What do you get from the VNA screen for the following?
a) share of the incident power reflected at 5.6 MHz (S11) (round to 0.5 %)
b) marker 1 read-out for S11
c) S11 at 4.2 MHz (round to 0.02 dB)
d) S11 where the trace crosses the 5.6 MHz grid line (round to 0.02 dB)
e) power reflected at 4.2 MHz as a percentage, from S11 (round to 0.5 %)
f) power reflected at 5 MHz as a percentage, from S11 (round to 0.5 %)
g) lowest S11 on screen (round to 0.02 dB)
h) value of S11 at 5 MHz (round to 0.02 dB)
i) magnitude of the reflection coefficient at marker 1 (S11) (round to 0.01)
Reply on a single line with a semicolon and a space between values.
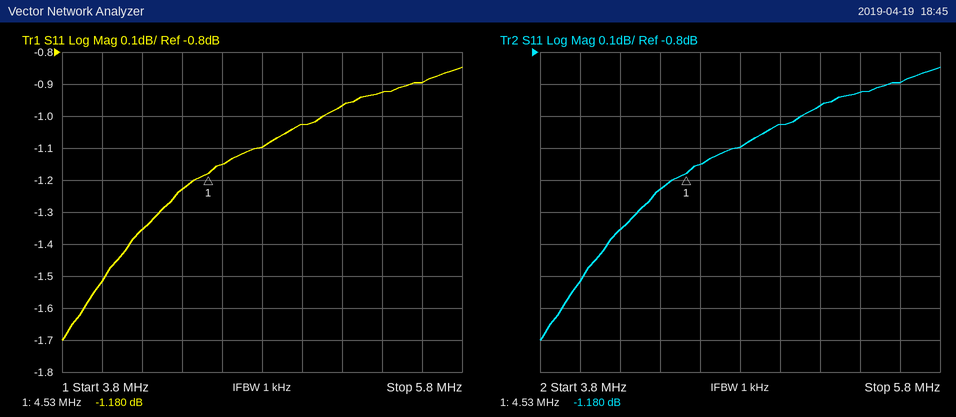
81.5 %; -1.180 dB; -1.36 dB; -0.90 dB; 73.0 %; 79.0 %; -1.70 dB; -1.02 dB; 0.87
